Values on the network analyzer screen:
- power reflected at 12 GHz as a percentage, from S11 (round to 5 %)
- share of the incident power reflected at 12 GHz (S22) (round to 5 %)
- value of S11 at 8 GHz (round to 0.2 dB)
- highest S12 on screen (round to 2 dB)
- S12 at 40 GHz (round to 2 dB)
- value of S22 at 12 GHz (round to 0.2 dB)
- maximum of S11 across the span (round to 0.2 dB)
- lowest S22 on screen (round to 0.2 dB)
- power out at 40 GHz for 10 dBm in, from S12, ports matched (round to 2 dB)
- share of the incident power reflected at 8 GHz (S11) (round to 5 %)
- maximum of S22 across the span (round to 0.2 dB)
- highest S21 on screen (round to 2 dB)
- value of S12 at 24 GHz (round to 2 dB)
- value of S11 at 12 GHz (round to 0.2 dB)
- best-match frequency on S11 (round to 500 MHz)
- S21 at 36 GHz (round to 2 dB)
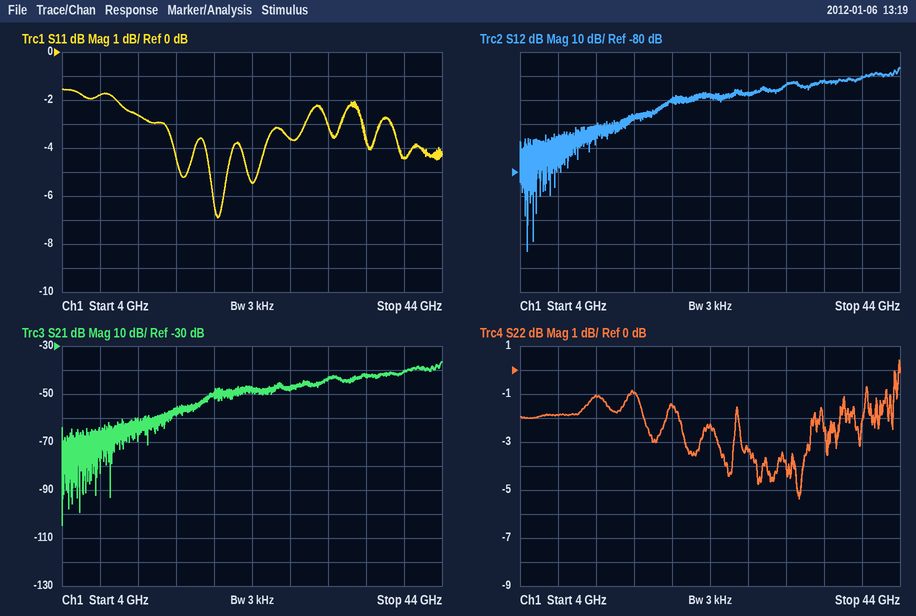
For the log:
55 %
80 %
-1.8 dB
-36 dB
-40 dB
-1.0 dB
-1.6 dB
-5.4 dB
-30 dBm
65 %
0.4 dB
-36 dB
-48 dB
-2.6 dB
20.5 GHz
-42 dB
